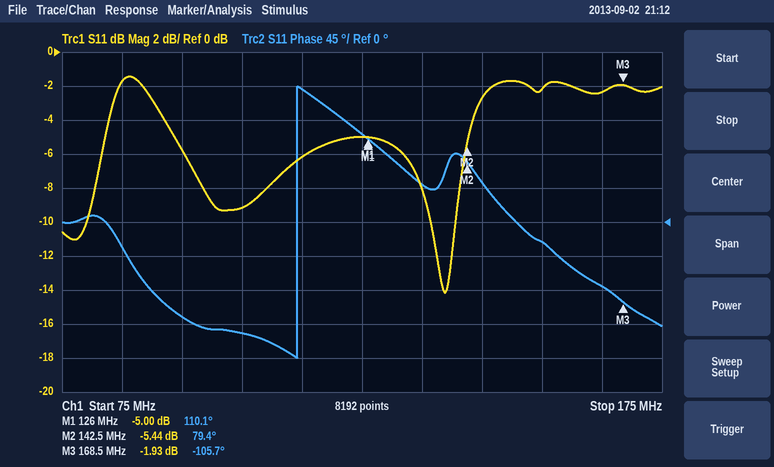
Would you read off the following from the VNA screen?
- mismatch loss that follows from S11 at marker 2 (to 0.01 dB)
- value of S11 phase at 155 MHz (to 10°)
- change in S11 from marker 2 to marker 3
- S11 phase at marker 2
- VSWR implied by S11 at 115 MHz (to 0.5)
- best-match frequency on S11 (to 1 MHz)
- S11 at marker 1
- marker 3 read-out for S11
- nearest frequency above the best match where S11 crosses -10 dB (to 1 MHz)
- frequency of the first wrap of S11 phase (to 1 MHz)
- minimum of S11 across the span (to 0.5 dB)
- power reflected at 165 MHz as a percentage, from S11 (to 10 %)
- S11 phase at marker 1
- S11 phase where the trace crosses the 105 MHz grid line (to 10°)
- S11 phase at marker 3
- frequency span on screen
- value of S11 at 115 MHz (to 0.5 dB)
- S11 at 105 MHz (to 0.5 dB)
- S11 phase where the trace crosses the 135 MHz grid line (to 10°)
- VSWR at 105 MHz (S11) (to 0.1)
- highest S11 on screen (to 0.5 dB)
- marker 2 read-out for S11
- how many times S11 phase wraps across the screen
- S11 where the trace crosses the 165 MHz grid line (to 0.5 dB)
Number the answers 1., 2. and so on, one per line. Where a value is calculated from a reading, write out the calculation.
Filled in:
1. −10 log10(1 − 10^(-5.44/10)) ≈ 1.46 dB
2. -30°
3. -1.93 − (-5.44) = 3.51 dB
4. 79.4°
5. |Γ| = 10^(-6/20) = 0.5012; VSWR = (1 + 0.5012)/(1 − 0.5012) ≈ 3.0
6. 139 MHz
7. -5.00 dB
8. -1.93 dB
9. 141 MHz
10. 114 MHz
11. -14.0 dB
12. 10^(-2.5/10) ≈ 56.2 %, so 60 % to the nearest 10 %
13. 110.1°
14. -150°
15. -105.7°
16. 100 MHz
17. -6.0 dB
18. -9.0 dB
19. 50°
20. |Γ| = 10^(-9/20) = 0.3548; VSWR = (1 + 0.3548)/(1 − 0.3548) ≈ 2.1
21. -1.5 dB
22. -5.44 dB
23. 1
24. -2.5 dB
